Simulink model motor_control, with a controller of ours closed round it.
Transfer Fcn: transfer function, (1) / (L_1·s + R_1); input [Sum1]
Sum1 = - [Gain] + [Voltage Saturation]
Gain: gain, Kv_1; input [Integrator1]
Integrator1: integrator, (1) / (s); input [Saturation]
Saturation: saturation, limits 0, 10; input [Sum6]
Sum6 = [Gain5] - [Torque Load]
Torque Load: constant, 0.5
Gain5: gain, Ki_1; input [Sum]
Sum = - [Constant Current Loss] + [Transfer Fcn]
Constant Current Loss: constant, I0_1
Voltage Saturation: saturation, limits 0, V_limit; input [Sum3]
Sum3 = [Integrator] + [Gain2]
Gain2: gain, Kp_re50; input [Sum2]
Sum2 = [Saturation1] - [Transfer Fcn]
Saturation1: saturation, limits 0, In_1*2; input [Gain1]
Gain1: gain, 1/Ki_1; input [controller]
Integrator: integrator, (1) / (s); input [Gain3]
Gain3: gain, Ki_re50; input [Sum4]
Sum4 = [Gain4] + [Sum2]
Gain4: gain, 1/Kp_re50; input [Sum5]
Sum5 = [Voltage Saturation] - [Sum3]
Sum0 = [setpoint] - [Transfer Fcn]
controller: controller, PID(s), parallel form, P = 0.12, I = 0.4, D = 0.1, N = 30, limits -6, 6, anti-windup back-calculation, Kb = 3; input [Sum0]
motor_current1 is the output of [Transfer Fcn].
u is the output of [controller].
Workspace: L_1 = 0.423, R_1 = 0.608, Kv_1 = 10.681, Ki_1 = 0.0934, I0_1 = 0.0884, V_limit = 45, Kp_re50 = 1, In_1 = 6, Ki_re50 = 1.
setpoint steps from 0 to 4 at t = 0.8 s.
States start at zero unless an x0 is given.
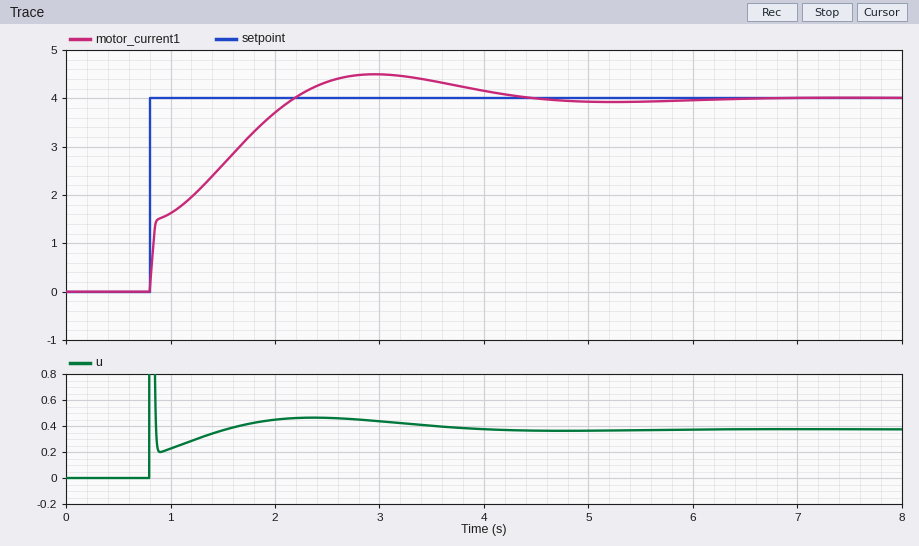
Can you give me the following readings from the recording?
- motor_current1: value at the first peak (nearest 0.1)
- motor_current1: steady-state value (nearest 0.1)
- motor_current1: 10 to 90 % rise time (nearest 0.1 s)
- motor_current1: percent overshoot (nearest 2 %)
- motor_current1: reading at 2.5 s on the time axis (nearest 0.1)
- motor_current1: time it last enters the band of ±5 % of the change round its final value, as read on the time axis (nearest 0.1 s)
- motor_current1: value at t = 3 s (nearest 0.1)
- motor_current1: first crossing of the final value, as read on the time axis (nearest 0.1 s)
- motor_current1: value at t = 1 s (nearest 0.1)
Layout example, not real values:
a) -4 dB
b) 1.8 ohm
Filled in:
a) 4.5
b) 4.0
c) 1.1 s
d) 12 %
e) 4.3
f) 3.9 s
g) 4.5
h) 2.2 s
i) 1.6
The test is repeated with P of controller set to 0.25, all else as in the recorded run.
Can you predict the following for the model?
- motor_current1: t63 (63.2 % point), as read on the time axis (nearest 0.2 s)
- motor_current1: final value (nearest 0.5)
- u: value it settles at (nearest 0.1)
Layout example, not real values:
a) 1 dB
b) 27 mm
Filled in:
a) 1.2 s
b) 4.0
c) 0.4
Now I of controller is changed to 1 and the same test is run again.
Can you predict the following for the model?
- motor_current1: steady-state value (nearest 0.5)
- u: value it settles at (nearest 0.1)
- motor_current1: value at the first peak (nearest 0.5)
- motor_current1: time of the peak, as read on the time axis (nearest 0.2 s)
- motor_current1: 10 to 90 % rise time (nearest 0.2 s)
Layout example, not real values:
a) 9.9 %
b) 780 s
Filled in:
a) 4.0
b) 0.4
c) 5.0
d) 2.0 s
e) 0.6 s
